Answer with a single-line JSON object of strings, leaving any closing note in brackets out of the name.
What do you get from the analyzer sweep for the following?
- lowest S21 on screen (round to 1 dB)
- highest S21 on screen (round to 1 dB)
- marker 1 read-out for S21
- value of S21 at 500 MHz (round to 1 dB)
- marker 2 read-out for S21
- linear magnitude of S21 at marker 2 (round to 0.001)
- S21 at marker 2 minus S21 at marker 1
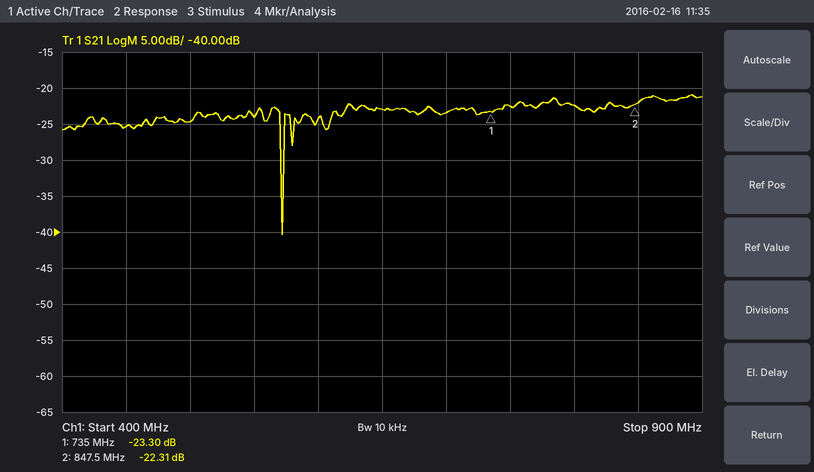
{"lowest S21 on screen": "-40 dB", "highest S21 on screen": "-21 dB", "marker 1 read-out for S21": "-23.30 dB", "value of S21 at 500 MHz": "-25 dB", "marker 2 read-out for S21": "-22.31 dB", "linear magnitude of S21 at marker 2": "0.077", "S21 at marker 2 minus S21 at marker 1": "0.99 dB"}
